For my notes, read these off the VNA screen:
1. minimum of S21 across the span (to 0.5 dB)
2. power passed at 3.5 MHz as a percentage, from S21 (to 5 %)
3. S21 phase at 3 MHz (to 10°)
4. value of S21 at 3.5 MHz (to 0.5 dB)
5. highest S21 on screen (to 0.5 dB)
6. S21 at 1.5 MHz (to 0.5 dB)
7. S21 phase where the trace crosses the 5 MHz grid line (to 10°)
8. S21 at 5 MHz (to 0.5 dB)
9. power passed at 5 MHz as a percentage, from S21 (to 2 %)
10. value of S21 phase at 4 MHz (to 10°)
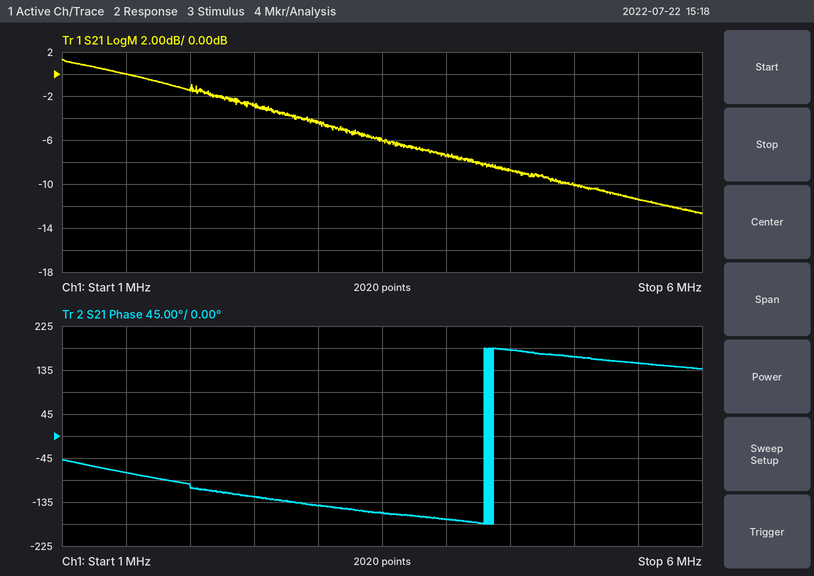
-12.5 dB
25 %
-140°
-6.0 dB
1.5 dB
0.0 dB
160°
-10.0 dB
10 %
-170°
